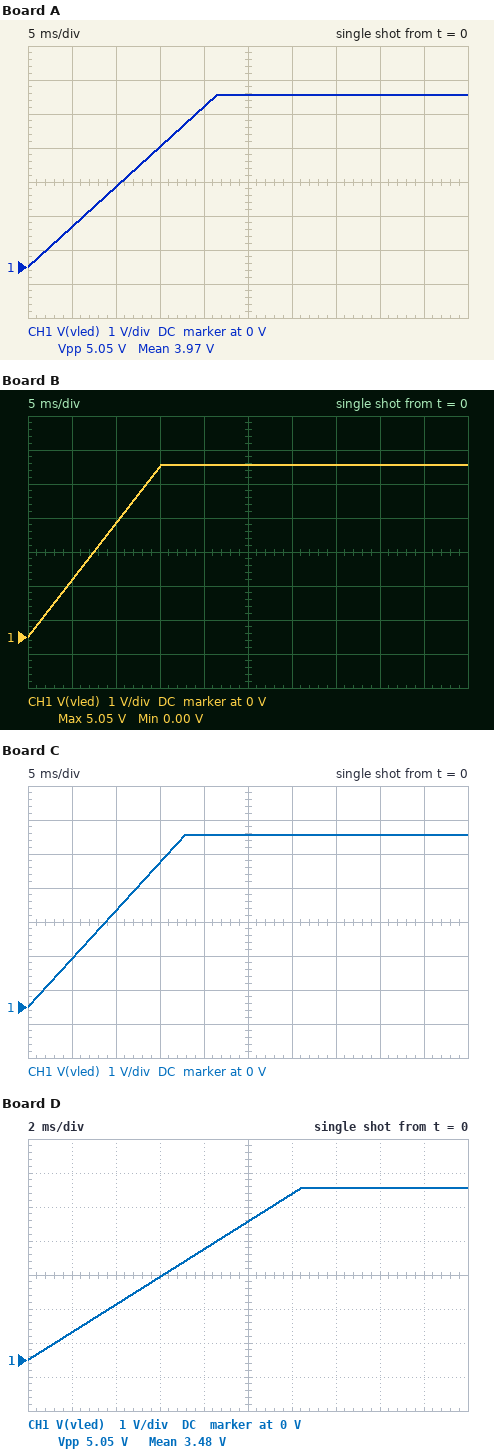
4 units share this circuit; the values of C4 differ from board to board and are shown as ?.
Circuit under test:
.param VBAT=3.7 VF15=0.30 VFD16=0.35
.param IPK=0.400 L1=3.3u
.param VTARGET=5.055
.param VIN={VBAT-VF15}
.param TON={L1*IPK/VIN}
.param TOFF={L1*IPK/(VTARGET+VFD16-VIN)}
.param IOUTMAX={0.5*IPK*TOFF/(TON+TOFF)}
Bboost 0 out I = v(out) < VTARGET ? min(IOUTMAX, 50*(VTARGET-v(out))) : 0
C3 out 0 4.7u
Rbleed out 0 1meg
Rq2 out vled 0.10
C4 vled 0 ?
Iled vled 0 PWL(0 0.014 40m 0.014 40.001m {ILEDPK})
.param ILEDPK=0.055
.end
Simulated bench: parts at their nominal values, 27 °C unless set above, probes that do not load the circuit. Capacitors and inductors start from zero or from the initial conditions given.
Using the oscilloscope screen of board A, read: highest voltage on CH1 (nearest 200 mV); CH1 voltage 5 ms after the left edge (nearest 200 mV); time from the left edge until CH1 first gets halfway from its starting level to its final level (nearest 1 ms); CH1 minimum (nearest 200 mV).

5.0 V
1.2 V
11 ms
0 V
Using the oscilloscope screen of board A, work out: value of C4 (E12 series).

470 µF
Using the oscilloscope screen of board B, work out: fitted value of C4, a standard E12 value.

330 µF
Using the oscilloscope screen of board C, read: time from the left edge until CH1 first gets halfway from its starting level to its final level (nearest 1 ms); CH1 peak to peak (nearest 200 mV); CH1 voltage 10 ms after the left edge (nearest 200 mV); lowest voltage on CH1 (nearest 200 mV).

9 ms
5.0 V
2.8 V
0 V
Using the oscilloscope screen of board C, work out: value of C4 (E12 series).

390 µF
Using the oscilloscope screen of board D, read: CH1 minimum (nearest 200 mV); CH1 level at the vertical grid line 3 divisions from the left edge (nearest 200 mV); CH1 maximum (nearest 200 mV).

0 V
2.4 V
5.0 V
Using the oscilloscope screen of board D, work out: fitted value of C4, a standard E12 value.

270 µF
